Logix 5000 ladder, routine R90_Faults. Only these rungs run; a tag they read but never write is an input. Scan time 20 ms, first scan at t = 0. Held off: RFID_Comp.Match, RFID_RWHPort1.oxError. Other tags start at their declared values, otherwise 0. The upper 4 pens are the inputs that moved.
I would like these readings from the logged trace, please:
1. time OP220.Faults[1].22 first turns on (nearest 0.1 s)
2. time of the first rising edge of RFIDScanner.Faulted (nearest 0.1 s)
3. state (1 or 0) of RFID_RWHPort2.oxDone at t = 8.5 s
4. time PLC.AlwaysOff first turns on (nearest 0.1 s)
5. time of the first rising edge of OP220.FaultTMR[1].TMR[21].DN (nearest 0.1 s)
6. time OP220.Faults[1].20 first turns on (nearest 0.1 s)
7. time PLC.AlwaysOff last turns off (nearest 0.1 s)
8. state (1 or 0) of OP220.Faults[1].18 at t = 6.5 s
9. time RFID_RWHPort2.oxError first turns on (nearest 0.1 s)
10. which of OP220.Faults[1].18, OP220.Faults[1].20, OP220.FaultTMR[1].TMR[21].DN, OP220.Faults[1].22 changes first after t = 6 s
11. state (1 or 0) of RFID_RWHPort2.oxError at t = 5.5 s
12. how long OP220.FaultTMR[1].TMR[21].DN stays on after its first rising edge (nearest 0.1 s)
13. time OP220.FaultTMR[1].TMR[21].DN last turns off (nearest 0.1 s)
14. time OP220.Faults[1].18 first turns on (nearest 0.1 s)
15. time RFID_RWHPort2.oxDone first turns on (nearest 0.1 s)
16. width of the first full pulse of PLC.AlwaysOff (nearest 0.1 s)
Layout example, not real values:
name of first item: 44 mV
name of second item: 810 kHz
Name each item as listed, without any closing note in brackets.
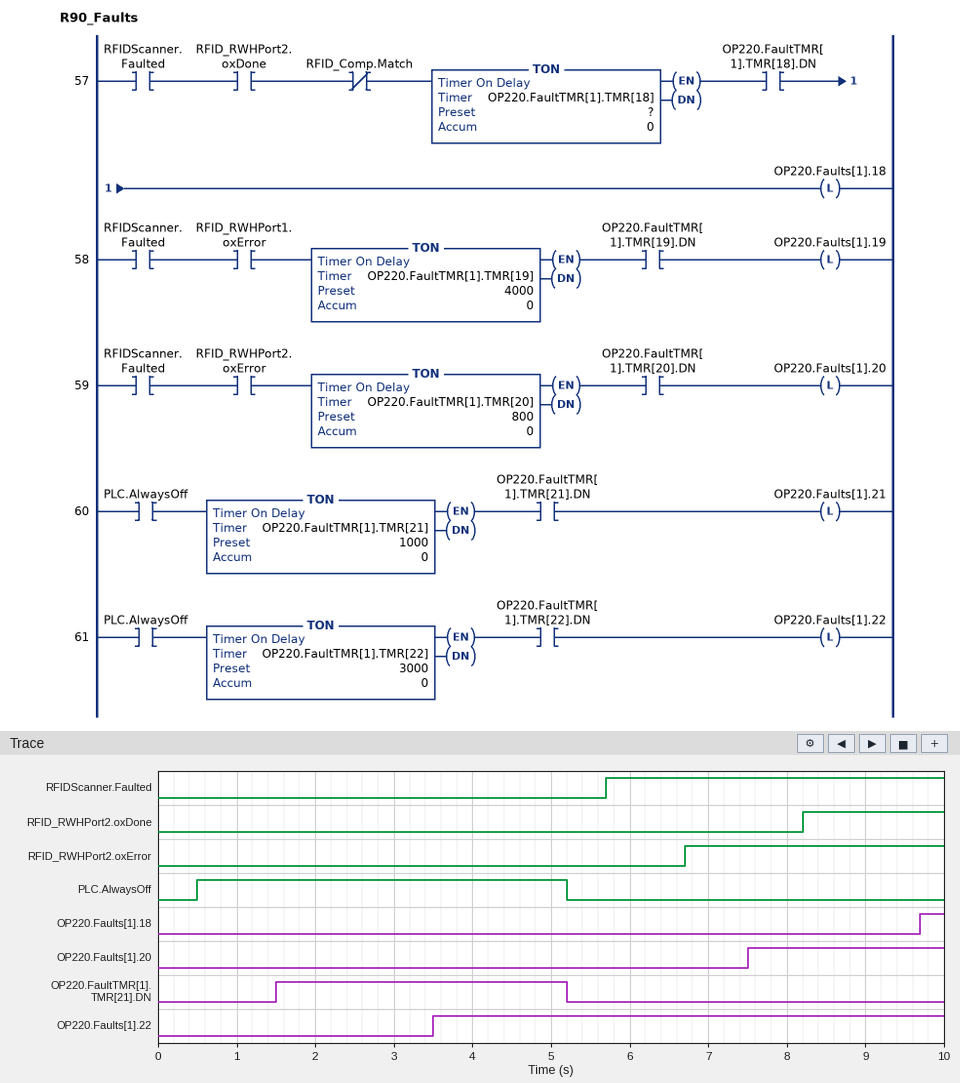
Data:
time OP220.Faults[1].22 first turns on: 3.5 s
time of the first rising edge of RFIDScanner.Faulted: 5.7 s
state (1 or 0) of RFID_RWHPort2.oxDone at t = 8.5 s: 1
time PLC.AlwaysOff first turns on: 0.5 s
time of the first rising edge of OP220.FaultTMR[1].TMR[21].DN: 1.5 s
time OP220.Faults[1].20 first turns on: 7.5 s
time PLC.AlwaysOff last turns off: 5.2 s
state (1 or 0) of OP220.Faults[1].18 at t = 6.5 s: 0
time RFID_RWHPort2.oxError first turns on: 6.7 s
which of OP220.Faults[1].18, OP220.Faults[1].20, OP220.FaultTMR[1].TMR[21].DN, OP220.Faults[1].22 changes first after t = 6 s: OP220.Faults[1].20
state (1 or 0) of RFID_RWHPort2.oxError at t = 5.5 s: 0
how long OP220.FaultTMR[1].TMR[21].DN stays on after its first rising edge: 3.7 s
time OP220.FaultTMR[1].TMR[21].DN last turns off: 5.2 s
time OP220.Faults[1].18 first turns on: 9.7 s
time RFID_RWHPort2.oxDone first turns on: 8.2 s
width of the first full pulse of PLC.AlwaysOff: 4.7 s
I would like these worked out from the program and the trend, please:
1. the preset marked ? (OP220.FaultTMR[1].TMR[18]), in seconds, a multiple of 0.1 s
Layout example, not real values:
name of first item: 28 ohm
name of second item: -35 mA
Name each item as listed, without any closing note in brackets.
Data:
the preset marked ? (OP220.FaultTMR[1].TMR[18]), in seconds, a multiple of 0.1 s: 1.5 s
